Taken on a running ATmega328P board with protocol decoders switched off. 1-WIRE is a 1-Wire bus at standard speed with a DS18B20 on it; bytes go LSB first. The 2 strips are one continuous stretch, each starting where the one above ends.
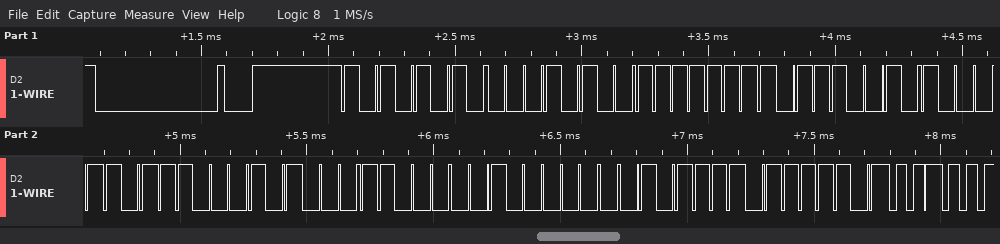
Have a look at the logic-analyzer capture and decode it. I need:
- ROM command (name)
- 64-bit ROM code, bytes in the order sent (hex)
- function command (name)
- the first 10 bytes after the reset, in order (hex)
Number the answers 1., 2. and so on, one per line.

1. Match ROM
2. 28 FF 4E B1 A3 18 04 F4
3. Read Scratchpad
4. 55 28 FF 4E B1 A3 18 04 F4 BE
